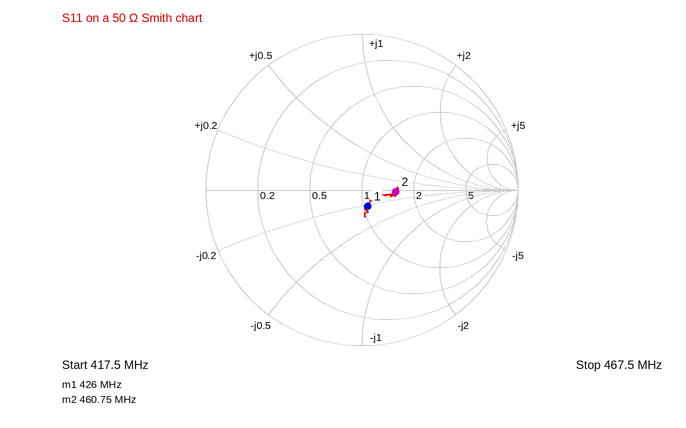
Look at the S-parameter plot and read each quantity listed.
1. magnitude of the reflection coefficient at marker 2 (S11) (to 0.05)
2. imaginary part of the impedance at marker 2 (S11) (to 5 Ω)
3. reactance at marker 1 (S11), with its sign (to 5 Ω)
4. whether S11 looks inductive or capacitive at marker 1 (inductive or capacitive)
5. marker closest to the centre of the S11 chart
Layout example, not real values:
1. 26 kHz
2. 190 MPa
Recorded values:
1. 0.20
2. 0 Ω
3. -10 Ω
4. capacitive
5. marker 1
